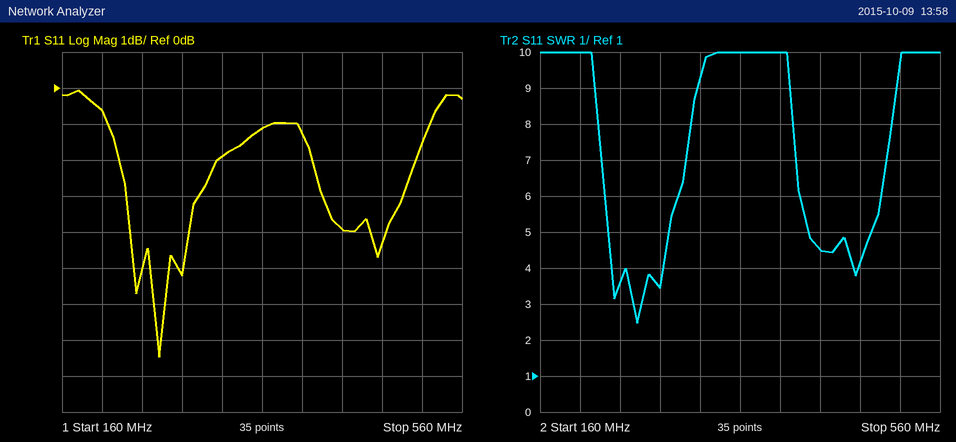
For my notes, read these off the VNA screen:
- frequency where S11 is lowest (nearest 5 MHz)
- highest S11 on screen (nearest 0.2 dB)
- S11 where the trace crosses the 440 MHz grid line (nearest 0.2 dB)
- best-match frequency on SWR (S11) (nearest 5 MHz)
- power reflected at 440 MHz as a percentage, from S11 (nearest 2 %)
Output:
255 MHz
0.0 dB
-4.0 dB
255 MHz
40 %
